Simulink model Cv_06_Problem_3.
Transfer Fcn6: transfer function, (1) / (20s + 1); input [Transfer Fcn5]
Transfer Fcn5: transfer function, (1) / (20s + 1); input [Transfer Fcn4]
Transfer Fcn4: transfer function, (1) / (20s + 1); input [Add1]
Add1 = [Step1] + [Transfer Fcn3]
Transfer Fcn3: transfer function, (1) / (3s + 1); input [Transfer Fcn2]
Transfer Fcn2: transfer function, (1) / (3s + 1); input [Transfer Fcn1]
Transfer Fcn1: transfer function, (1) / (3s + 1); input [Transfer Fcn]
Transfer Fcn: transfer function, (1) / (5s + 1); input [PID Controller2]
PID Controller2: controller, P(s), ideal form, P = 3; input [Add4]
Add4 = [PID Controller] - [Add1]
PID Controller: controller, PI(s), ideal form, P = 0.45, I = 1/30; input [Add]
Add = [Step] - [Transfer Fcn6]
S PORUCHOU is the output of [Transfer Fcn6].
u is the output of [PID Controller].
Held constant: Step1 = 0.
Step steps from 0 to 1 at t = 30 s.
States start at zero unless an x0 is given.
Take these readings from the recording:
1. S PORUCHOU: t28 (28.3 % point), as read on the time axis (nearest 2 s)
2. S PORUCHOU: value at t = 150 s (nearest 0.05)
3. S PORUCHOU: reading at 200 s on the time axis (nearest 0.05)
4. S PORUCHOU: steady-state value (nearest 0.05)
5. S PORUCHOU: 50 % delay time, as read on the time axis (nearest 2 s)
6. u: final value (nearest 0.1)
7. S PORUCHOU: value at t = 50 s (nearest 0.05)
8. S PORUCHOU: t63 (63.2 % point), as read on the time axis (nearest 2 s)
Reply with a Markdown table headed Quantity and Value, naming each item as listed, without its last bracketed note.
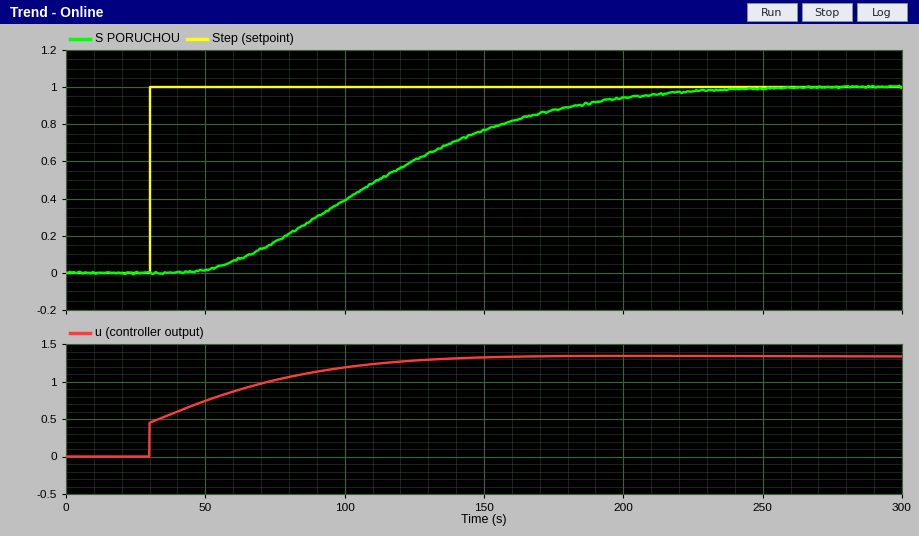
| Quantity | Value |
|---|---|
| S PORUCHOU: t28 (28.3 % point), as read on the time axis | 88 s |
| S PORUCHOU: value at t = 150 s | 0.75 |
| S PORUCHOU: reading at 200 s on the time axis | 0.95 |
| S PORUCHOU: steady-state value | 1.00 |
| S PORUCHOU: 50 % delay time, as read on the time axis | 112 s |
| u: final value | 1.3 |
| S PORUCHOU: value at t = 50 s | 0.00 |
| S PORUCHOU: t63 (63.2 % point), as read on the time axis | 128 s |
